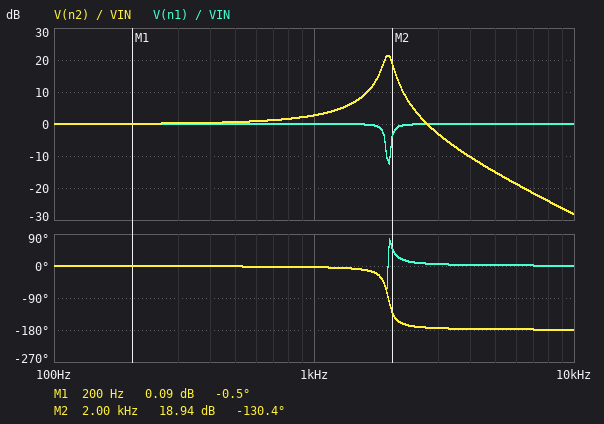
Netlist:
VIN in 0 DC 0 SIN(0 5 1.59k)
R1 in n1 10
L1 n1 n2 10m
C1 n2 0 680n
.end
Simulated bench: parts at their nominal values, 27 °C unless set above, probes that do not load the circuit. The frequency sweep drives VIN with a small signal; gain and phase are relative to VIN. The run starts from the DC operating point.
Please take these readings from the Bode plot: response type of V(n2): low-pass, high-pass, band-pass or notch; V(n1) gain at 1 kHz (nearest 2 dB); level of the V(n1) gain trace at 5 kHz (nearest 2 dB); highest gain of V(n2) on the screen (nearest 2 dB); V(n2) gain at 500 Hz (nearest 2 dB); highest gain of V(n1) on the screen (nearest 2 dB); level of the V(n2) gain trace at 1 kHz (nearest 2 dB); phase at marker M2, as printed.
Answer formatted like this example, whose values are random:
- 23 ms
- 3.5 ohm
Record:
- band-pass
- 0 dB
- 0 dB
- 22 dB
- 0 dB
- 0 dB
- 2 dB
- -130.4 deg
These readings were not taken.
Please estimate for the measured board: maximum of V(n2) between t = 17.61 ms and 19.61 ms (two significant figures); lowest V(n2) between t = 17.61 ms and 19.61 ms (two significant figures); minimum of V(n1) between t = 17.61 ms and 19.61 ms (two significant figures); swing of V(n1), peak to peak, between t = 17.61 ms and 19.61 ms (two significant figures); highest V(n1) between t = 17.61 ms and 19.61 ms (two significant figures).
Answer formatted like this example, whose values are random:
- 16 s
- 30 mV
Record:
- 15 V
- -15 V
- -4.9 V
- 9.8 V
- 4.9 V
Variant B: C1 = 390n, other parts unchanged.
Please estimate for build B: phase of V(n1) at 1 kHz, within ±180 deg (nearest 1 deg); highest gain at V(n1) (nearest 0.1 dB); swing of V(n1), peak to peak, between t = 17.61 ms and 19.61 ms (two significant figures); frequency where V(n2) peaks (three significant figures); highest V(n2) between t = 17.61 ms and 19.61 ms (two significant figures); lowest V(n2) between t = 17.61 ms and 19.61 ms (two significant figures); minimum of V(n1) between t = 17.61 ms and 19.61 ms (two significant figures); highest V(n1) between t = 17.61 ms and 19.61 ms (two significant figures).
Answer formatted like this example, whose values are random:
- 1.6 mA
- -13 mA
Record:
- -2 deg
- 0 dB
- 10 V
- 2.55 kHz
- 8.2 V
- -8.2 V
- -5.0 V
- 5.0 V
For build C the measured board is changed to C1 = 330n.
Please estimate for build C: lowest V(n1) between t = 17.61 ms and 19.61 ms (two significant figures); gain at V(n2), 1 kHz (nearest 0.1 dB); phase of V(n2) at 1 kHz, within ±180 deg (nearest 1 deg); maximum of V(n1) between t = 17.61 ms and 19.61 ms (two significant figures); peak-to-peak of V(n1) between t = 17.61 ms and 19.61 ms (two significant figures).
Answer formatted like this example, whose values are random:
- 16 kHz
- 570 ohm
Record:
- -5.0 V
- 1.2 dB
- -1 deg
- 5.0 V
- 10 V
